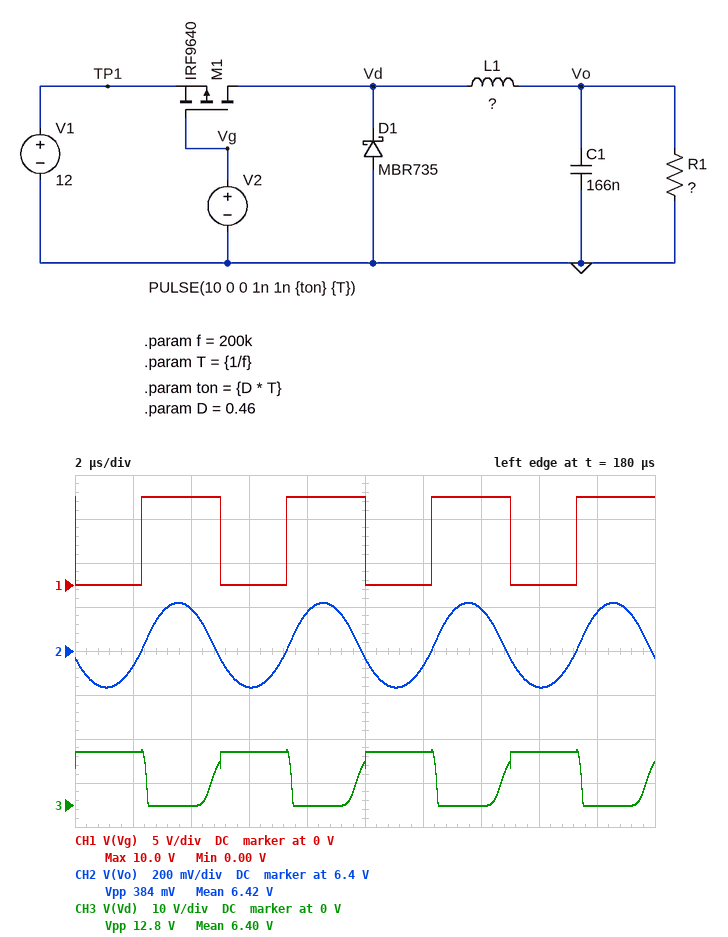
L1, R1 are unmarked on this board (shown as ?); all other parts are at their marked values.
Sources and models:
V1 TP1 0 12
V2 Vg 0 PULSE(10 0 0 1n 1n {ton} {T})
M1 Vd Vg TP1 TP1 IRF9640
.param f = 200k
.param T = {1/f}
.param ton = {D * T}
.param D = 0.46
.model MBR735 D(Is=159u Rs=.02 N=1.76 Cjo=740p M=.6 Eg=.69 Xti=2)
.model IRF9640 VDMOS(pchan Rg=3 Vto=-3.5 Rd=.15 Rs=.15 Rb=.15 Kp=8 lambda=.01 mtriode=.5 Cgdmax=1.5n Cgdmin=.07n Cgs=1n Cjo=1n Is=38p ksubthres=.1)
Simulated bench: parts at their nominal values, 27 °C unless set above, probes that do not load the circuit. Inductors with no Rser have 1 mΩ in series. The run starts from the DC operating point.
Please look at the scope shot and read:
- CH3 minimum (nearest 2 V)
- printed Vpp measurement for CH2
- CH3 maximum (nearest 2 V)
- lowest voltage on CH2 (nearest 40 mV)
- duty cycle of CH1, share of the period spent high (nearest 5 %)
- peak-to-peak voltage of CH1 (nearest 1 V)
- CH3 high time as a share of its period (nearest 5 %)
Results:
0 V
384 mV
12 V
6.24 V
55 %
10 V
55 %
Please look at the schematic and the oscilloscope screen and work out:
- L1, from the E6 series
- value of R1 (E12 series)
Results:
150 µH
220 Ω
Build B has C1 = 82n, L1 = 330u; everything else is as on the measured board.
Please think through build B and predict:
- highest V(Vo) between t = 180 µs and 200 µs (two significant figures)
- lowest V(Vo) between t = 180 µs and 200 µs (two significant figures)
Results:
6.1 V
5.8 V
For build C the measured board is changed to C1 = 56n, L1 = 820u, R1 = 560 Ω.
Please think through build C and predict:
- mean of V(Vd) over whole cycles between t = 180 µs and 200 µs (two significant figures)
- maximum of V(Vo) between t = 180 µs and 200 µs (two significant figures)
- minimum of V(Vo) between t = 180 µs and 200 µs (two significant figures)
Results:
6.7 V
6.8 V
6.6 V
